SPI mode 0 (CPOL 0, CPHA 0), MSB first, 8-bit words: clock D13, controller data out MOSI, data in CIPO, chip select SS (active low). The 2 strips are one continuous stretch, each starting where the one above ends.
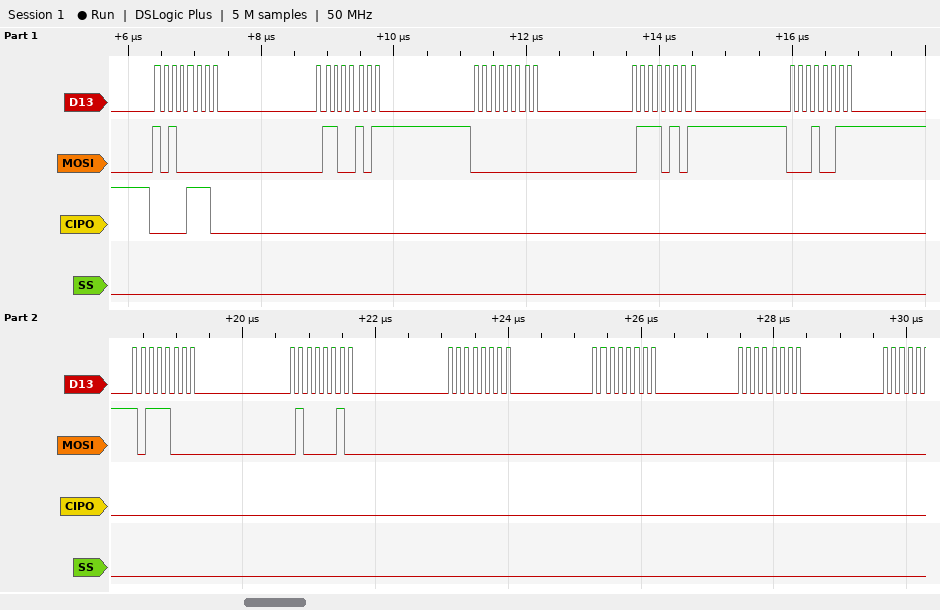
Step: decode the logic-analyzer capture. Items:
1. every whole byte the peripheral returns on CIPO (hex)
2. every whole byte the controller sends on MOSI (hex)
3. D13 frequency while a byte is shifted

0E 00 00 00 00 00 00 00 00 00
A0 65 00 75 13 B8 42 00 00 00
8 MHz
